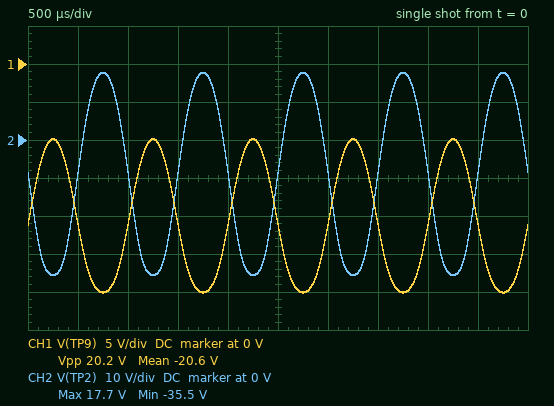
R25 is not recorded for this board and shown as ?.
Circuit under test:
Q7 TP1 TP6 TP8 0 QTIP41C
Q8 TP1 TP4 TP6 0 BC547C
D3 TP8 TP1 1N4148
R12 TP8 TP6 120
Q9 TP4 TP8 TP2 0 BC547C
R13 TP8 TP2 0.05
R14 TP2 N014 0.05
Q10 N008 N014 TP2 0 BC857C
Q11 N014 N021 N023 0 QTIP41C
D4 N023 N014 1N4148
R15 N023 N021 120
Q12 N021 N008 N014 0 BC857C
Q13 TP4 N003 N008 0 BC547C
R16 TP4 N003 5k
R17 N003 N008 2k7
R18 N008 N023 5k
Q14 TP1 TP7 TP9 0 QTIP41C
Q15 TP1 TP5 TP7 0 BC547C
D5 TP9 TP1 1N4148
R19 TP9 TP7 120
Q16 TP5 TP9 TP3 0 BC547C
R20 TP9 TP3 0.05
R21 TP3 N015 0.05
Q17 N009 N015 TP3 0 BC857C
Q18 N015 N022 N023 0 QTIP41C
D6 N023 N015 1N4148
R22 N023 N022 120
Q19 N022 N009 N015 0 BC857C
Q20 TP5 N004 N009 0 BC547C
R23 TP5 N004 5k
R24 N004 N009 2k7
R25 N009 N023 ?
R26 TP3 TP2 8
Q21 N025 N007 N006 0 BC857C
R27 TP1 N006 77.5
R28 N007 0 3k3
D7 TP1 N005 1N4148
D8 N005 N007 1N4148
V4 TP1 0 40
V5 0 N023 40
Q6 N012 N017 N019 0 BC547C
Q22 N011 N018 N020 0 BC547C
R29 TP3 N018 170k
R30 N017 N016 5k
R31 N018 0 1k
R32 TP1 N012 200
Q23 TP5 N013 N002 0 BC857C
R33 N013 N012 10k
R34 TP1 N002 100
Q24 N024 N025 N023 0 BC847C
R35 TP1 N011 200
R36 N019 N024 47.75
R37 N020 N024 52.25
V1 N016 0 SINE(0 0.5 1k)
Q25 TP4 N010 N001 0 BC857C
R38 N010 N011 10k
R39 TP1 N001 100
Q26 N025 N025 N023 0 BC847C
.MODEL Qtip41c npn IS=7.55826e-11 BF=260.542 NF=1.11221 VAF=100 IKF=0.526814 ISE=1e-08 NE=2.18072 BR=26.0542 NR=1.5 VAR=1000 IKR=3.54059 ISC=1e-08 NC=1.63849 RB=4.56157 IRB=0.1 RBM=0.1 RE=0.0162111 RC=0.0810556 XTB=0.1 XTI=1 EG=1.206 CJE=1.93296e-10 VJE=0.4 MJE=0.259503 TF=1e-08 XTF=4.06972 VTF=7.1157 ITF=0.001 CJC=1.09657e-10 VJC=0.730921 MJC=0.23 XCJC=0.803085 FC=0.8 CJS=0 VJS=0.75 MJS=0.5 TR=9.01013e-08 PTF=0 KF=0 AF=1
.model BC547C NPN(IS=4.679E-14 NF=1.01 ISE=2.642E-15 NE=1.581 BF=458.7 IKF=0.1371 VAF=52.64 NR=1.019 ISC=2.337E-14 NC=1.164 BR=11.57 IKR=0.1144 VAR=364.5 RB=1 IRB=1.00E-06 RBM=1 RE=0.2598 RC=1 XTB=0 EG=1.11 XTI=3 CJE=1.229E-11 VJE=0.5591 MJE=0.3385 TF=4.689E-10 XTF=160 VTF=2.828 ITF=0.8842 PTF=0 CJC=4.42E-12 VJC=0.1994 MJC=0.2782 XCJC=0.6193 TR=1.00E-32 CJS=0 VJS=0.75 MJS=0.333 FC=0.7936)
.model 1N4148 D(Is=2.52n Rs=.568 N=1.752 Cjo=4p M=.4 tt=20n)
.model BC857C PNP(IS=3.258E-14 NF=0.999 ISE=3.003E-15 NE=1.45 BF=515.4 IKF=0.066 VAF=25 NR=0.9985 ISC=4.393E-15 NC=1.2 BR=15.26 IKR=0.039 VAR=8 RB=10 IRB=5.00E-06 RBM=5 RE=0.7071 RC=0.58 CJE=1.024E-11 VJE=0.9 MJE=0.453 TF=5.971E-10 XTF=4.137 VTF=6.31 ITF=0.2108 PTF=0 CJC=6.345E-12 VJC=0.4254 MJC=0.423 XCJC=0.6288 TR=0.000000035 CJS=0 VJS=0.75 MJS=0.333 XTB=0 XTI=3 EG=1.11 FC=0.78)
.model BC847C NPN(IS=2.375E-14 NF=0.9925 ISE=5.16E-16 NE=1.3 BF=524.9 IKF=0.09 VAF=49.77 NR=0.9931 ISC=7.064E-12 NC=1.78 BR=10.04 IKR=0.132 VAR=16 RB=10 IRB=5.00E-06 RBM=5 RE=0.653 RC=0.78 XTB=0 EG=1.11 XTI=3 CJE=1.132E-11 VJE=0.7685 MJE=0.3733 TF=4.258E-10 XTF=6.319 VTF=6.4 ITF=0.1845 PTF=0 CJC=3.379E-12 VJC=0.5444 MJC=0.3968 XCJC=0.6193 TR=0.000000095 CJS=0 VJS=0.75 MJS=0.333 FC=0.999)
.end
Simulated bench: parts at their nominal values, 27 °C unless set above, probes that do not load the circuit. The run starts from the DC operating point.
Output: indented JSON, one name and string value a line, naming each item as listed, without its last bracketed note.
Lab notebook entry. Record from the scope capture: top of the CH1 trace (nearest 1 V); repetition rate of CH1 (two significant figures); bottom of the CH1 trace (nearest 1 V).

{
  "top of the CH1 trace": "-10 V",
  "repetition rate of CH1": "1.0 kHz",
  "bottom of the CH1 trace": "-30 V"
}
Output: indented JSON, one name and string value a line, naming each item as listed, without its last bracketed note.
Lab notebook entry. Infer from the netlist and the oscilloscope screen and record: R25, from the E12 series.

{
  "R25, from the E12 series": "1.8 kΩ"
}
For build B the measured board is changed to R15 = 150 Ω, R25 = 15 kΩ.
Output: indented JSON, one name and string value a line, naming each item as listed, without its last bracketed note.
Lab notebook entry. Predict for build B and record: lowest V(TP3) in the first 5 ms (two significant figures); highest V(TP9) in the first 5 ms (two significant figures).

{
  "lowest V(TP3) in the first 5 ms": "-12 V",
  "highest V(TP9) in the first 5 ms": "37 V"
}
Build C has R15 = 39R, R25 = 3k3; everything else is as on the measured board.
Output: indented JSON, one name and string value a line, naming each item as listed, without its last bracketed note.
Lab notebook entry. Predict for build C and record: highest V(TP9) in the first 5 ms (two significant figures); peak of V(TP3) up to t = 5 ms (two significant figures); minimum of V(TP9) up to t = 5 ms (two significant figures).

{
  "highest V(TP9) in the first 5 ms": "7.5 V",
  "peak of V(TP3) up to t = 5 ms": "7.3 V",
  "minimum of V(TP9) up to t = 5 ms": "-26 V"
}
